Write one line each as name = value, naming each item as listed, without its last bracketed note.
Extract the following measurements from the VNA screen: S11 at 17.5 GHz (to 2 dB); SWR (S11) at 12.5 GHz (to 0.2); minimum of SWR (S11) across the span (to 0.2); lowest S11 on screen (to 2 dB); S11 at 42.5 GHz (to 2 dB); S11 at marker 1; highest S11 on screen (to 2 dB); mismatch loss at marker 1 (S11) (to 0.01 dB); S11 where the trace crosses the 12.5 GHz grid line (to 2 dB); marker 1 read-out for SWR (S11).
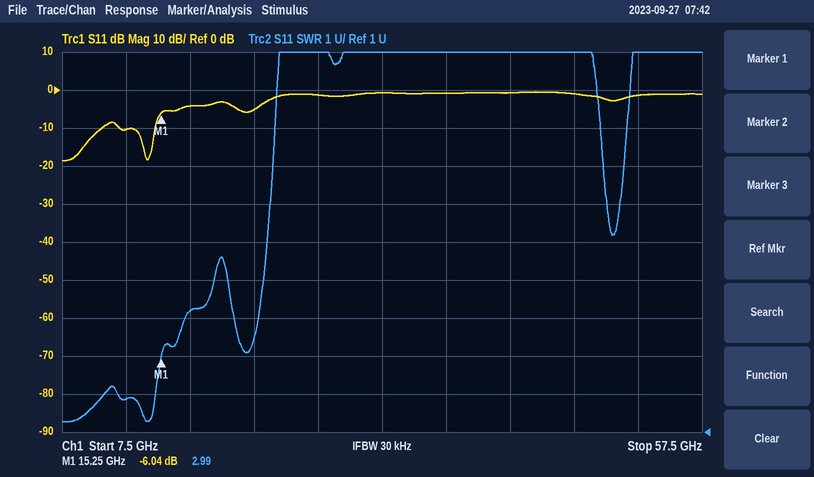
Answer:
S11 at 17.5 GHz = -4 dB
SWR (S11) at 12.5 GHz = 1.8
minimum of SWR (S11) across the span = 1.2
lowest S11 on screen = -18 dB
S11 at 42.5 GHz = 0 dB
S11 at marker 1 = -6.04 dB
highest S11 on screen = 0 dB
mismatch loss at marker 1 (S11) = 1.24 dB
S11 where the trace crosses the 12.5 GHz grid line = -10 dB
marker 1 read-out for SWR = 2.99
